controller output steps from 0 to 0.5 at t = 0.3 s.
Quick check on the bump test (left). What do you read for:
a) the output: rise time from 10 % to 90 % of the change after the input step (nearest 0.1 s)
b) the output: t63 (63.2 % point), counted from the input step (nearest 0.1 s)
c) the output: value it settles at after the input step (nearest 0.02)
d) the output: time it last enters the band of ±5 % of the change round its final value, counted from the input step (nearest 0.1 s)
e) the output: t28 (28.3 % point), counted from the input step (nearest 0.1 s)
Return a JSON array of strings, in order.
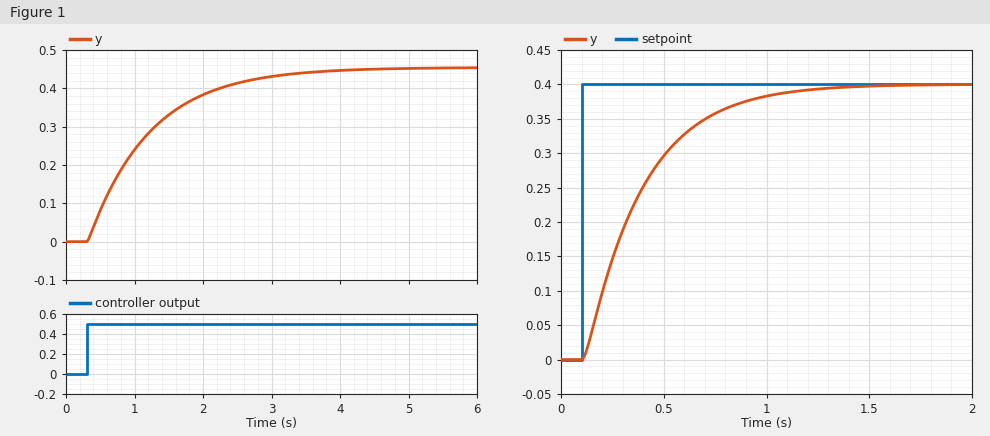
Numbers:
["2.0 s", "0.9 s", "0.46", "2.7 s", "0.3 s"]
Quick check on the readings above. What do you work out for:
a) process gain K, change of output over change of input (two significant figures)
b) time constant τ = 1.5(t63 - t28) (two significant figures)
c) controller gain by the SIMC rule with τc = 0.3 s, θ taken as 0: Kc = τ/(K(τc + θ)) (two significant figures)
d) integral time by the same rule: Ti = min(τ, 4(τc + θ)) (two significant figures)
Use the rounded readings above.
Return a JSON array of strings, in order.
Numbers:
["0.92", "0.90 s", "3.3", "0.90 s"]
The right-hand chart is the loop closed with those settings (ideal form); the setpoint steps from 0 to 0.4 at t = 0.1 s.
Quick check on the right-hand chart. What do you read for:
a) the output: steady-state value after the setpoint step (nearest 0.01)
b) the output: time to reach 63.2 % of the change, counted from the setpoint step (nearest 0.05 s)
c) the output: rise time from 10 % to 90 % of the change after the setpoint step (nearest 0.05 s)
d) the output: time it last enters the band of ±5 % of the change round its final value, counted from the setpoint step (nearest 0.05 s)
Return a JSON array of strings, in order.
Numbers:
["0.40", "0.30 s", "0.60 s", "0.85 s"]
